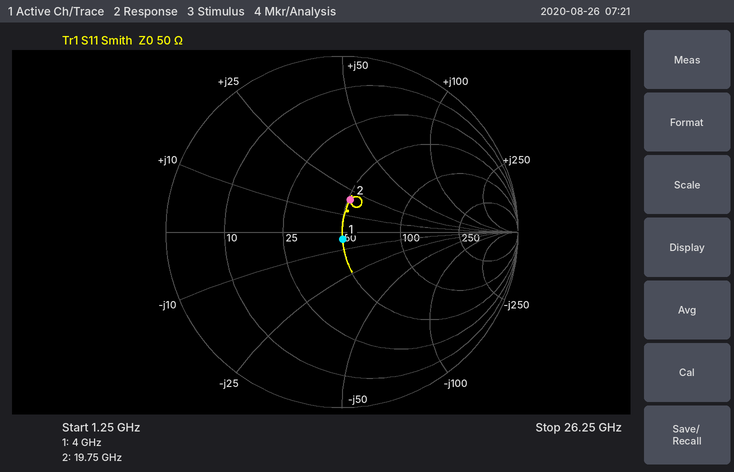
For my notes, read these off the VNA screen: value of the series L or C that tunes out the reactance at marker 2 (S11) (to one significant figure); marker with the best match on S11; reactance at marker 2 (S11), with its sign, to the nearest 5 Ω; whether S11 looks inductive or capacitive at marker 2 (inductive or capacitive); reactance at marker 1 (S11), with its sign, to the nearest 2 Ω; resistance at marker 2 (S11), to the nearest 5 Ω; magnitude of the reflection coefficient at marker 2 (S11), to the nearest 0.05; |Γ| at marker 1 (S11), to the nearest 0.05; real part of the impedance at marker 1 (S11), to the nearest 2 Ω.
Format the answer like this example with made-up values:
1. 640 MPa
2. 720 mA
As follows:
1. 400 fF
2. marker 1
3. +20 Ω
4. inductive
5. -4 Ω
6. 50 Ω
7. 0.20
8. 0.05
9. 50 Ω
